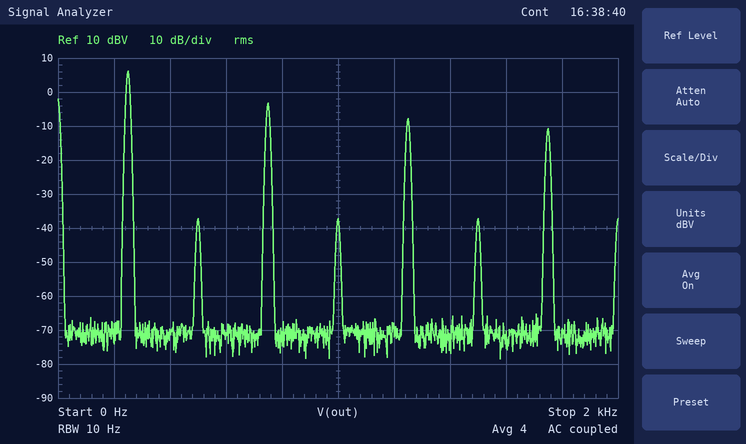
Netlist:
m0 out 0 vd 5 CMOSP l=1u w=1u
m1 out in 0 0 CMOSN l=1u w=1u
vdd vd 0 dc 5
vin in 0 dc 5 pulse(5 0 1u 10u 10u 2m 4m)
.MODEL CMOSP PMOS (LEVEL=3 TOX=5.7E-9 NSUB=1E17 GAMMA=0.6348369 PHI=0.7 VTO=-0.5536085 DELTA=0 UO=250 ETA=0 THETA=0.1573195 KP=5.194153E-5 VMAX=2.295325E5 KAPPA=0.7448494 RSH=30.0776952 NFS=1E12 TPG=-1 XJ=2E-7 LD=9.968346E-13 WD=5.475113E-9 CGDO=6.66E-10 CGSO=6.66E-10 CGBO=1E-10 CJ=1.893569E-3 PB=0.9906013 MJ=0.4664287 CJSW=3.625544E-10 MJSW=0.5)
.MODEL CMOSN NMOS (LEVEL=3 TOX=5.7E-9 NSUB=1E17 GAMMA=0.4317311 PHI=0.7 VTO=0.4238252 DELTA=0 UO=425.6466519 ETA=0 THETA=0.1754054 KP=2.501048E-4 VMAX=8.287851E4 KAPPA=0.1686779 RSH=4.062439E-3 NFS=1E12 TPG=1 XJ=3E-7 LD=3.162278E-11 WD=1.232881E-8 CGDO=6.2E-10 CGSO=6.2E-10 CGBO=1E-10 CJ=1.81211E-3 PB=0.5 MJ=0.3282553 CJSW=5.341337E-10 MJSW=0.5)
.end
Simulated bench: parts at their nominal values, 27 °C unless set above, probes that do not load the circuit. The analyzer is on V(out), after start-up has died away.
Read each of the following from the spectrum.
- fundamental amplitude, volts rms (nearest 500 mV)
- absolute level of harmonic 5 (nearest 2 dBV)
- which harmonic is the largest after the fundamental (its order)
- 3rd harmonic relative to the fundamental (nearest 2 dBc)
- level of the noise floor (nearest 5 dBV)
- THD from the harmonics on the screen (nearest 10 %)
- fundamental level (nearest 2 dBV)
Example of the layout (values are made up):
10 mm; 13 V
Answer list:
2.0 V; -8 dBV; 3; -10 dBc; -70 dBV; 40 %; 6 dBV
